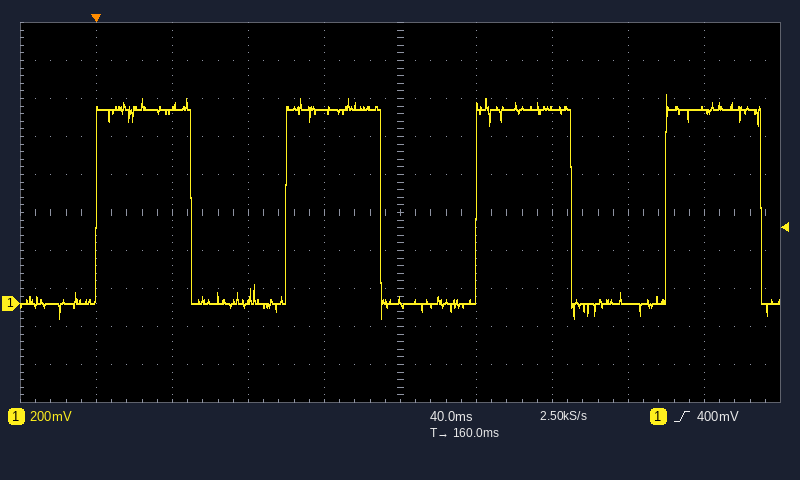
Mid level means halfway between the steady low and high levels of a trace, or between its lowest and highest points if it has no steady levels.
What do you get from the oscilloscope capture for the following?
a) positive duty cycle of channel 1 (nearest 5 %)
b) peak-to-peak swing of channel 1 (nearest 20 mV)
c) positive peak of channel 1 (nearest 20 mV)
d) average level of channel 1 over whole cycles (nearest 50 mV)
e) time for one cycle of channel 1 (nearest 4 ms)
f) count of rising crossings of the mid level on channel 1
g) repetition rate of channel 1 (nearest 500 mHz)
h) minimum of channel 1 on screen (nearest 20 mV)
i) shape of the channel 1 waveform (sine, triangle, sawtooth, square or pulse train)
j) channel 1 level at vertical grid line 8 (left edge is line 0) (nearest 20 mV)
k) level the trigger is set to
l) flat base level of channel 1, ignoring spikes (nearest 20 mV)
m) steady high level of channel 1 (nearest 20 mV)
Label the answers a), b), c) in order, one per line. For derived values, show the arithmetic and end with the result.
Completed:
a) 50 %
b) 1.10 V − (-80 mV) = 1.18 V
c) 1.10 V
d) 0 mV + 0.5 × (1.02 V − (0 mV)) ≈ 510 mV, so 500 mV to the nearest 50 mV
e) 100 ms
f) 4
g) 1 / 100 ms ≈ 10.0 Hz
h) -80 mV
i) square
j) 0 mV
k) 400 mV
l) 0 mV
m) 1.02 V
